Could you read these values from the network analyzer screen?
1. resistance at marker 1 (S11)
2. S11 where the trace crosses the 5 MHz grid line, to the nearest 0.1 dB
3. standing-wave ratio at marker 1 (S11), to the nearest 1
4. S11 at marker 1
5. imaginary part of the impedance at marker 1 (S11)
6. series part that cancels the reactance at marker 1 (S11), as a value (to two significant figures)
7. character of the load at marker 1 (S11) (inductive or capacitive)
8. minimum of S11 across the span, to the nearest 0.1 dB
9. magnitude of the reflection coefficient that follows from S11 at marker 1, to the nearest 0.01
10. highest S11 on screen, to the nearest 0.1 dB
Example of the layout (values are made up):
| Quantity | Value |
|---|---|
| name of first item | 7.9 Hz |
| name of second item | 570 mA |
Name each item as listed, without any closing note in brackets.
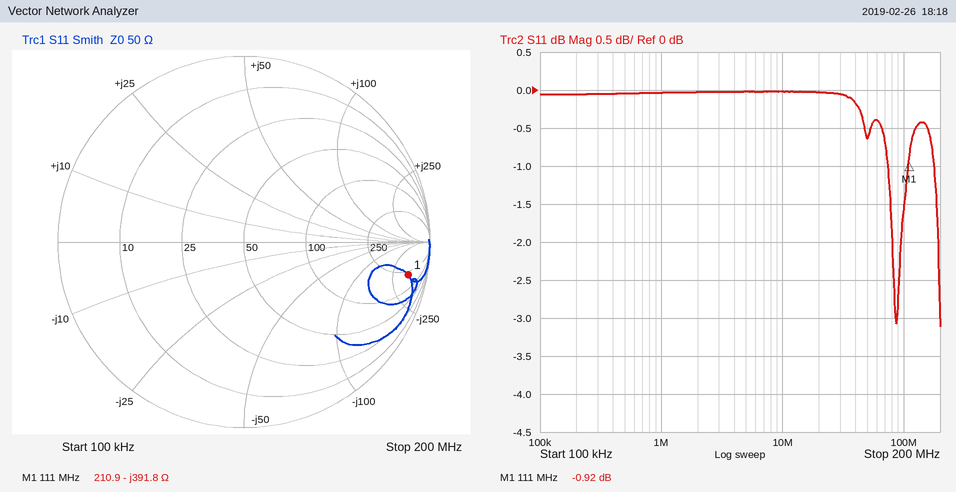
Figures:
| Quantity | Value |
|---|---|
| resistance at marker 1 | 210.9 Ω |
| S11 where the trace crosses the 5 MHz grid line, to the nearest 0.1 dB | 0.0 dB |
| standing-wave ratio at marker 1 (S11), to the nearest 1 | 19 |
| S11 at marker 1 | -0.92 dB |
| imaginary part of the impedance at marker 1 | -391.8 Ω |
| series part that cancels the reactance at marker 1 (S11), as a value | 560 nH |
| character of the load at marker 1 (S11) | capacitive |
| minimum of S11 across the span, to the nearest 0.1 dB | -3.1 dB |
| magnitude of the reflection coefficient that follows from S11 at marker 1, to the nearest 0.01 | 0.90 |
| highest S11 on screen, to the nearest 0.1 dB | 0.0 dB |
